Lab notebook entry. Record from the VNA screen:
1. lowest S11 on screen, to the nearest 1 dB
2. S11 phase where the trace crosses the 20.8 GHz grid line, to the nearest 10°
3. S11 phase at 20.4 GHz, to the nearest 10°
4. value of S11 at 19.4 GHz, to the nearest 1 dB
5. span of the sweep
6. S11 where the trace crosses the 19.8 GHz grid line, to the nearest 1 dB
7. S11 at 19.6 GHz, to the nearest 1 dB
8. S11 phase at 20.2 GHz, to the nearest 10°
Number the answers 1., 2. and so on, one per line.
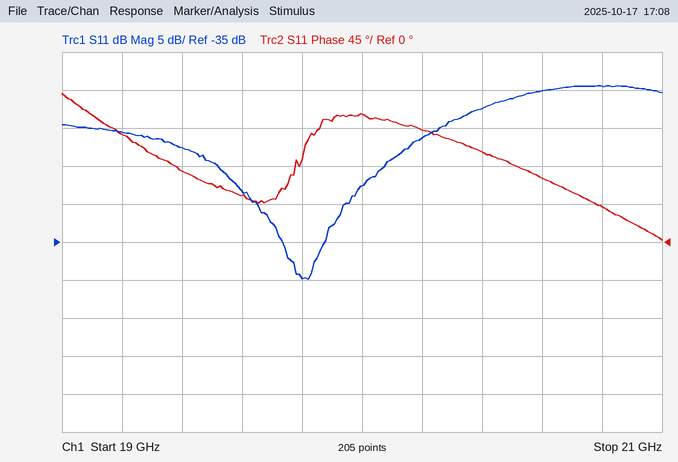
1. -40 dB
2. 40°
3. 110°
4. -23 dB
5. 2 GHz
6. -40 dB
7. -28 dB
8. 130°
